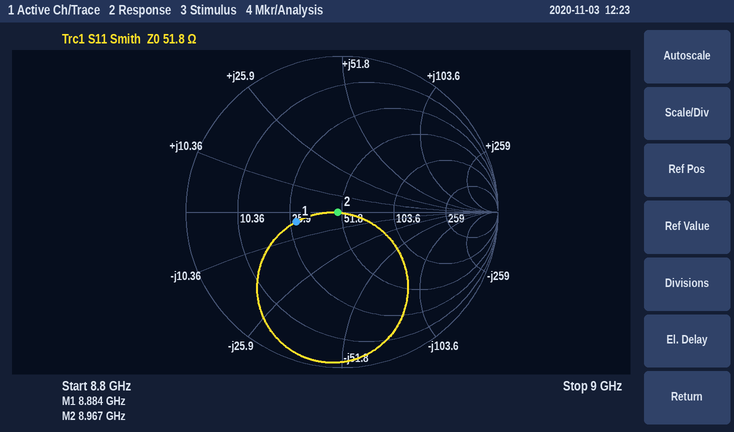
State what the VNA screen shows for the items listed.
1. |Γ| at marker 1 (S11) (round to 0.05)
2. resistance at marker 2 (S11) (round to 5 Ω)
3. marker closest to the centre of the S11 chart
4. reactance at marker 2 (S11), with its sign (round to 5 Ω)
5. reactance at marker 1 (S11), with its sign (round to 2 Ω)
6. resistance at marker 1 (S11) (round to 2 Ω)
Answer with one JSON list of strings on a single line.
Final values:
["0.30", "50 Ω", "marker 2", "0 Ω", "-4 Ω", "28 Ω"]
